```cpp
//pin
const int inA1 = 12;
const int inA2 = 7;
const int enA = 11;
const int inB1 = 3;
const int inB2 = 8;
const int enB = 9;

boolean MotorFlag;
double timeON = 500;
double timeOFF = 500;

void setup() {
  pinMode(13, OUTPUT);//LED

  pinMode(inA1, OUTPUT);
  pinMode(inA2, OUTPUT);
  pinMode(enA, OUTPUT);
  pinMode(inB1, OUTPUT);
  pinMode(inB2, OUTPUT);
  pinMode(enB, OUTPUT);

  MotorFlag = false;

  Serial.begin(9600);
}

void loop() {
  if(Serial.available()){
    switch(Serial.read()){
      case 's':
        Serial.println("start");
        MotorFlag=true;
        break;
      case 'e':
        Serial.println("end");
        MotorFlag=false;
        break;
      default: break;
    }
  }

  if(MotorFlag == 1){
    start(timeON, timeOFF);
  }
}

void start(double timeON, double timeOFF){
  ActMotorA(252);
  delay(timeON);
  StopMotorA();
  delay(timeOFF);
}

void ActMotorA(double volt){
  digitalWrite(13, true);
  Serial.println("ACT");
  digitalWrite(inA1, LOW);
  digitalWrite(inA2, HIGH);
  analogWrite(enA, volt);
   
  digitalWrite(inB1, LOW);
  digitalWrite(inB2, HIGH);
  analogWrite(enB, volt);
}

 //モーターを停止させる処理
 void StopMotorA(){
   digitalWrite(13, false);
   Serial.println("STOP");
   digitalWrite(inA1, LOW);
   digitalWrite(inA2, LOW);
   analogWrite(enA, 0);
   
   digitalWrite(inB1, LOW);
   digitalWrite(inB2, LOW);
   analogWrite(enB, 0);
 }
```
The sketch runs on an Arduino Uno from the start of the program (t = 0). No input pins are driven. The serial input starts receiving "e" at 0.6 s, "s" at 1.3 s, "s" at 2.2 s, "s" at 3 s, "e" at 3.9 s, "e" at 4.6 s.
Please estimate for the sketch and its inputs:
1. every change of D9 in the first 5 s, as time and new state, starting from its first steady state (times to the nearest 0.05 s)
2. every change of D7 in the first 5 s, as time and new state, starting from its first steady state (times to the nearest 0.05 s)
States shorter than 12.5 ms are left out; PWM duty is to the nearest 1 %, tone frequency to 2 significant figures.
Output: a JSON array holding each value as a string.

["0 s low; 1.3 s PWM 99 %; 1.8 s low; 2.3 s PWM 99 %; 2.8 s low; 3.3 s PWM 99 %; 3.8 s low", "0 s low; 1.3 s high; 1.8 s low; 2.3 s high; 2.8 s low; 3.3 s high; 3.8 s low"]
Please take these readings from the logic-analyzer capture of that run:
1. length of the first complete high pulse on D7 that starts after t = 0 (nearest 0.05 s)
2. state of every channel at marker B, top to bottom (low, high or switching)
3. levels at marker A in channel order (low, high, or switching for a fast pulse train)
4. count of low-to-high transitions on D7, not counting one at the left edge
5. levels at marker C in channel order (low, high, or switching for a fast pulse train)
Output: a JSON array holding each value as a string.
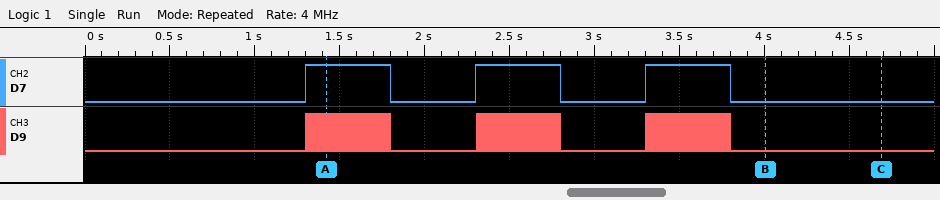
["0.50 s", "D7 low, D9 low", "D7 high, D9 switching", "3", "D7 low, D9 low"]
